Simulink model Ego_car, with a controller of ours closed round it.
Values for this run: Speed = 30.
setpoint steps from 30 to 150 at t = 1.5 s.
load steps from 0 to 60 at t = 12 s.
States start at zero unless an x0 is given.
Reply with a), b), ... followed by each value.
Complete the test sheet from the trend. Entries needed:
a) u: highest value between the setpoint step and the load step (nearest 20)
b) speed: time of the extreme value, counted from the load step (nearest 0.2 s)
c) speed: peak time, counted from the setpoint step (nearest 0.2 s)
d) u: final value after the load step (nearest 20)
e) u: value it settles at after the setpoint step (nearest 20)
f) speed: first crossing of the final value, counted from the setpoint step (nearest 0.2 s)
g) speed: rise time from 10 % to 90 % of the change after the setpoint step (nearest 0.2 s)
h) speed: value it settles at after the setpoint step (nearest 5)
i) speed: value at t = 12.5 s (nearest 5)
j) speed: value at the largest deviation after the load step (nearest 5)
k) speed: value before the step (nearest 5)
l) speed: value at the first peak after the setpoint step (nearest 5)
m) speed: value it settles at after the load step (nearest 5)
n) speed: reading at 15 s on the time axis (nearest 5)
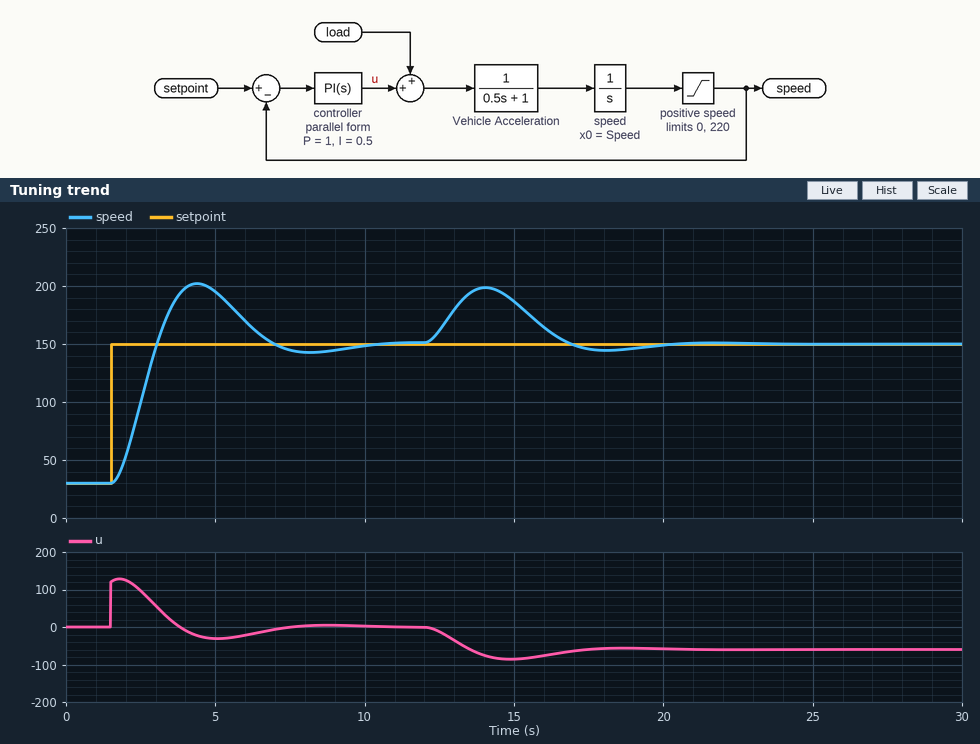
a) 120
b) 2.0 s
c) 2.8 s
d) -60
e) 0
f) 1.6 s
g) 1.0 s
h) 150
i) 160
j) 200
k) 30
l) 200
m) 150
n) 185
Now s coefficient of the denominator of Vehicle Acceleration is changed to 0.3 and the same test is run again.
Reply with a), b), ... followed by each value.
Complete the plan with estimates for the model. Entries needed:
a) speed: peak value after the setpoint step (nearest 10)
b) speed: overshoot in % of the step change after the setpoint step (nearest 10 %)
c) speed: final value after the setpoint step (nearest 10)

a) 190
b) 30 %
c) 150
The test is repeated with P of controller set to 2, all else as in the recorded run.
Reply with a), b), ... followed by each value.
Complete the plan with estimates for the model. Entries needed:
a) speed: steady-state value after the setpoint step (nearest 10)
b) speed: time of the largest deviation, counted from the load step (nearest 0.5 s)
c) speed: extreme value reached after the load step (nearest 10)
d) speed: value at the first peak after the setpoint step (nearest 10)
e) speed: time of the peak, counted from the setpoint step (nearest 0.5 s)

a) 150
b) 1.5 s
c) 180
d) 190
e) 2.0 s
